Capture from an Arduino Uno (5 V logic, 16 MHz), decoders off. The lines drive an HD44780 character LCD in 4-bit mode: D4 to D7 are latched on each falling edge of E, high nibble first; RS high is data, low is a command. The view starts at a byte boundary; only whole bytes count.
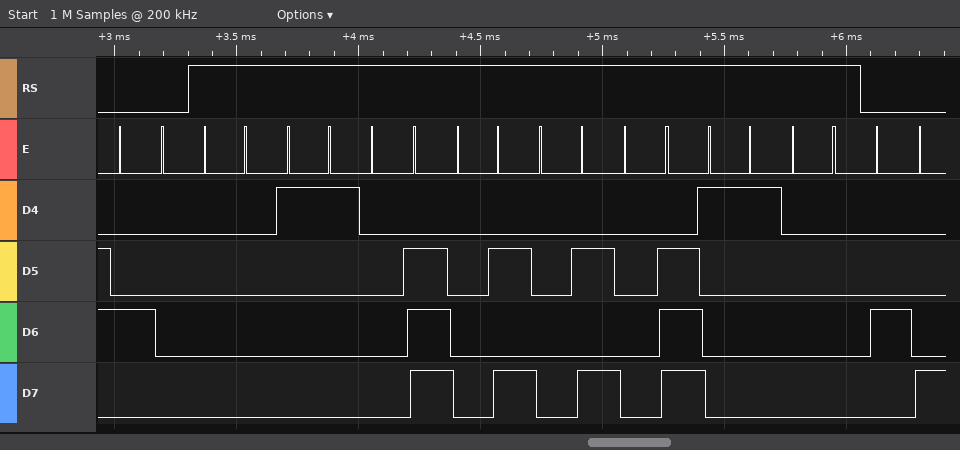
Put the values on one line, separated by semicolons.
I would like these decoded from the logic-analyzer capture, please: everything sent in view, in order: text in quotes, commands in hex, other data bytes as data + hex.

0x40 data 00 11 0E 0A 0A 0E 11 00 0x48
